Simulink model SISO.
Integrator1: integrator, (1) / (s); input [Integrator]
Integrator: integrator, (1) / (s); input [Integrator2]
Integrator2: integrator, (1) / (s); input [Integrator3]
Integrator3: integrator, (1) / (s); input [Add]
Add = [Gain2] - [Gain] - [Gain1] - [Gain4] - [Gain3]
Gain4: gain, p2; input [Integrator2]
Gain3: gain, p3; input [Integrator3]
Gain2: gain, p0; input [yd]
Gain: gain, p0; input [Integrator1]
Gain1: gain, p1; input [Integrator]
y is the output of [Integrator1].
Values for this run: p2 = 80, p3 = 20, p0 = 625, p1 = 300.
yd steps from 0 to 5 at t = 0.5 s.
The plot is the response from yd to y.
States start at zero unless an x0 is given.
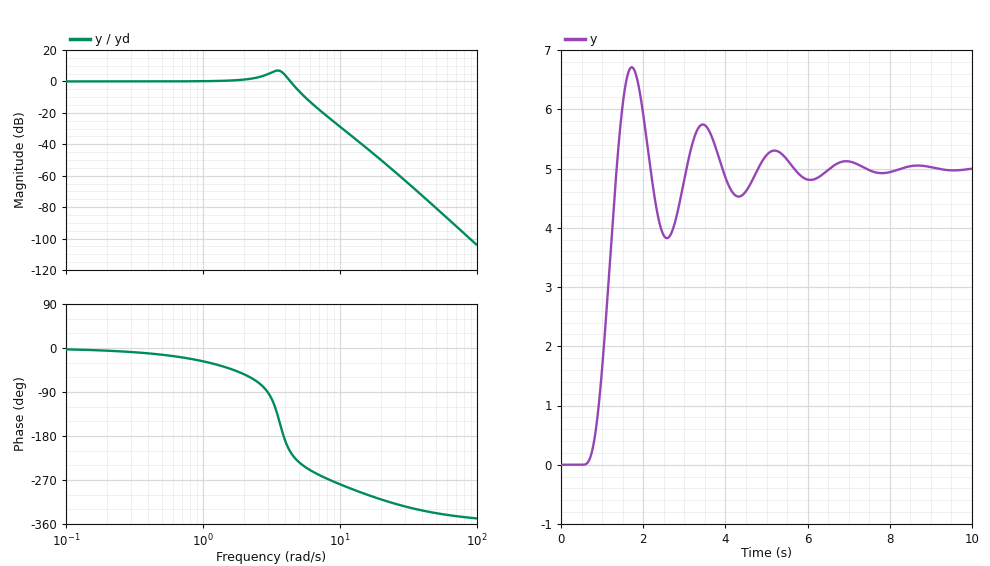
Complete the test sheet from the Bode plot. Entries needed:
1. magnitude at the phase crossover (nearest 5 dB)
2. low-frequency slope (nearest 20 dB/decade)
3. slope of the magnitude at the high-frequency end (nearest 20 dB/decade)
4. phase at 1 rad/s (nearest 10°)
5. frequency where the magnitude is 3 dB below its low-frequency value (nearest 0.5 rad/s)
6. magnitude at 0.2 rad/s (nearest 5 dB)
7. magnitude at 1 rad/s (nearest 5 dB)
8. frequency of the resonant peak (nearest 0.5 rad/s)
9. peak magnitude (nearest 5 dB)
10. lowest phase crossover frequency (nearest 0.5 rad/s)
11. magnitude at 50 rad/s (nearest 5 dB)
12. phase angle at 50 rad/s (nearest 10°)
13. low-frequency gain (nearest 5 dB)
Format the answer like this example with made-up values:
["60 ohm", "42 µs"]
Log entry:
["5 dB", "0 dB/decade", "-80 dB/decade", "-30°", "4.5 rad/s", "0 dB", "0 dB", "3.5 rad/s", "5 dB", "4.0 rad/s", "-80 dB", "-340°", "0 dB"]
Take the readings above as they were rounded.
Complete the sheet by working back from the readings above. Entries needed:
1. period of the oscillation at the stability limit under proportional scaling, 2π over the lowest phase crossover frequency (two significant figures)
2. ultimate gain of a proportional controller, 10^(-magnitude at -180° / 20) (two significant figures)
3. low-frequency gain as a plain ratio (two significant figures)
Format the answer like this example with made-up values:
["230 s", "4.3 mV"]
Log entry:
["1.6 s", "0.56", "1.0"]
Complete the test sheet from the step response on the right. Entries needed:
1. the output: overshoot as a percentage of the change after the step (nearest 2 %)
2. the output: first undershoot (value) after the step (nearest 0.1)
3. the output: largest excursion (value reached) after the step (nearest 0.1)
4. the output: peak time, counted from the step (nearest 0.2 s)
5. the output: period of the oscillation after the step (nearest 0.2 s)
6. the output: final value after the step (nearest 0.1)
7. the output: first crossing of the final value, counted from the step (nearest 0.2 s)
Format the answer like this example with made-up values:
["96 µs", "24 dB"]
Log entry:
["34 %", "3.8", "6.7", "1.2 s", "1.8 s", "5.0", "0.8 s"]
